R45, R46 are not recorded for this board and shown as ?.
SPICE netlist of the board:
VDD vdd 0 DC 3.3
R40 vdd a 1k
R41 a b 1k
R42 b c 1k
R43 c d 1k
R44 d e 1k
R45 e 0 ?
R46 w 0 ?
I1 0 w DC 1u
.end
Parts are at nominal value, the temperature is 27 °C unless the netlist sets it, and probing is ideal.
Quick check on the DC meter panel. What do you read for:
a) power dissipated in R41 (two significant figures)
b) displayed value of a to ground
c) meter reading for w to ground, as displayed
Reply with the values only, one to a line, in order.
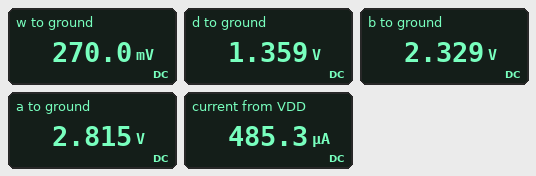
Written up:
240 µW
2.815 V
270.0 mV
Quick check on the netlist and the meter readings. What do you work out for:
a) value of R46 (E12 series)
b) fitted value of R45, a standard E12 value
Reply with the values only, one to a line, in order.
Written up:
270 kΩ
1.8 kΩ
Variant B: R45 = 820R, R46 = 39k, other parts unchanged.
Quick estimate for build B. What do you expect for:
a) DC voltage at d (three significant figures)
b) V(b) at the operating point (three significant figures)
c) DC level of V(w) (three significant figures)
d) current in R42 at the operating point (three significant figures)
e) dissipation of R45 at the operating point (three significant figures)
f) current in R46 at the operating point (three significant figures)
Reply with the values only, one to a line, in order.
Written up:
1.03 V
2.17 V
39.0 mV
567 µA
264 µW
1.00 µA
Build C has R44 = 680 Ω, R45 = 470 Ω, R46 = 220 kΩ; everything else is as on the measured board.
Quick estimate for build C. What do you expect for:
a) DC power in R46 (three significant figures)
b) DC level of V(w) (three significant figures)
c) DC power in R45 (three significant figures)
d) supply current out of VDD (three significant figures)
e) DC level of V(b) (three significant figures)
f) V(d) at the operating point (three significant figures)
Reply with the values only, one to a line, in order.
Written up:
220 nW
220 mV
193 µW
641 µA
2.02 V
737 mV
